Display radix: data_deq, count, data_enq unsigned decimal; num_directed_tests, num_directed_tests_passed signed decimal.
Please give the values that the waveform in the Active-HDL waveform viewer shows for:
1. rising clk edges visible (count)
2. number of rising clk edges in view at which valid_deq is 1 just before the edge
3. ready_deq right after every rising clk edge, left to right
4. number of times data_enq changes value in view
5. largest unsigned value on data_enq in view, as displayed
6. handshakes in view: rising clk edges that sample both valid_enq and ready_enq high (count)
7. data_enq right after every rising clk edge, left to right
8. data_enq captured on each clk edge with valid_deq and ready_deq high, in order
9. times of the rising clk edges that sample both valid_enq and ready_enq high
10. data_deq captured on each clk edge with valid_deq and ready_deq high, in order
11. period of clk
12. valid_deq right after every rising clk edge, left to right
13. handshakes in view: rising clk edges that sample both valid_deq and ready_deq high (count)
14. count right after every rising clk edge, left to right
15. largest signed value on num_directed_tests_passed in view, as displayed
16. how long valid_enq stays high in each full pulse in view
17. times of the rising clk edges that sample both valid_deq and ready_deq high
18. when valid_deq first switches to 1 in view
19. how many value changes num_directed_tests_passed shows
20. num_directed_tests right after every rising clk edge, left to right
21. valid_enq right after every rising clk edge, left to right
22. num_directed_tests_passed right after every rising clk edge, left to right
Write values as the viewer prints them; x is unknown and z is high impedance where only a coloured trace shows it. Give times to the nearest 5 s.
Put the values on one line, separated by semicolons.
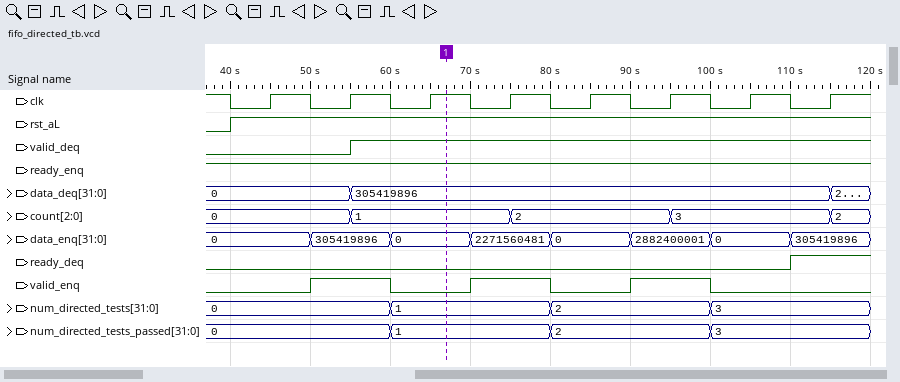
8; 6; 0 0 0 0 0 0 0 1; 7; 2882400001; 3; 0, 305419896, 0, 2271560481, 0, 2882400001, 0, 305419896; 305419896; 55 s, 75 s, 95 s; 305419896; 10 s; 0 1 1 1 1 1 1 1; 1; 0, 1, 1, 2, 2, 3, 3, 2; 3; 10 s, 10 s, 10 s; 115 s; 55 s; 3; 0, 0, 1, 1, 2, 2, 3, 3; 0 1 0 1 0 1 0 0; 0, 0, 1, 1, 2, 2, 3, 3
